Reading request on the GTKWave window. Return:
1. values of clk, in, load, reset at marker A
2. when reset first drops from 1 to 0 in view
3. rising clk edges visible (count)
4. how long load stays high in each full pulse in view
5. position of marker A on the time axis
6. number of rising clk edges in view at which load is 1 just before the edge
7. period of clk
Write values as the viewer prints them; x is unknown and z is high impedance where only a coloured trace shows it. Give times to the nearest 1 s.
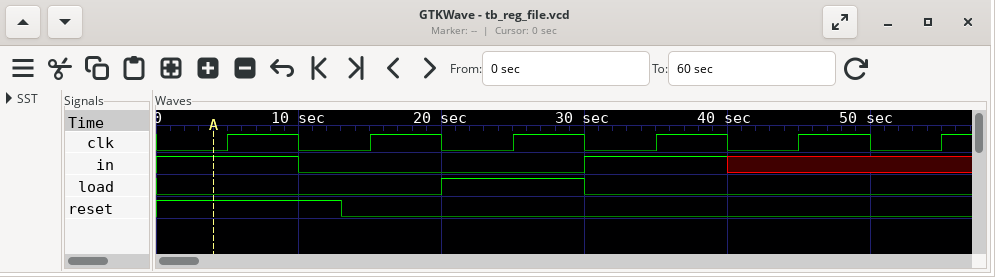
clk=0, in=1, load=0, reset=1
13 s
6
10 s
4 s
1
10 s
